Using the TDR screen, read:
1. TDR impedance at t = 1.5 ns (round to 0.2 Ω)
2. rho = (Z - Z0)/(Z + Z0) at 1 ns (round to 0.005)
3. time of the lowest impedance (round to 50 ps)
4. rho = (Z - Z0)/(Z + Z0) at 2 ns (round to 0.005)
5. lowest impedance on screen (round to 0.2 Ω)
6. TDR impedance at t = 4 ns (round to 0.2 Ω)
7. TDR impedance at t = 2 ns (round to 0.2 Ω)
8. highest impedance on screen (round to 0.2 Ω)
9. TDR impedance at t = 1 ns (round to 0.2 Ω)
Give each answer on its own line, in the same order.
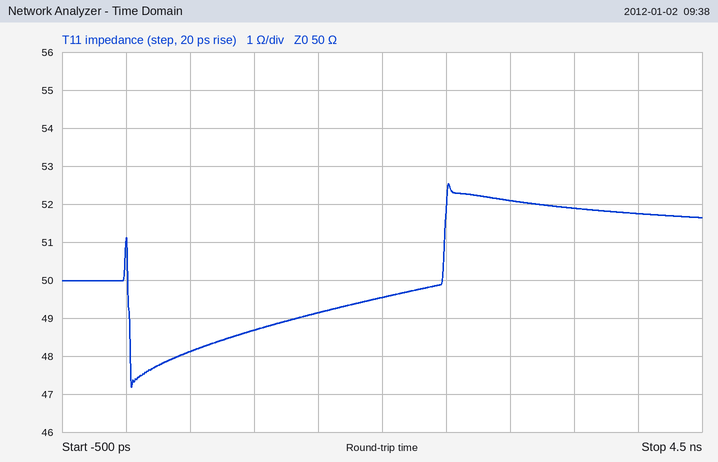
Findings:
49.2 Ω
-0.015
50 ps
-0.005
47.2 Ω
51.8 Ω
49.6 Ω
52.6 Ω
48.6 Ω
